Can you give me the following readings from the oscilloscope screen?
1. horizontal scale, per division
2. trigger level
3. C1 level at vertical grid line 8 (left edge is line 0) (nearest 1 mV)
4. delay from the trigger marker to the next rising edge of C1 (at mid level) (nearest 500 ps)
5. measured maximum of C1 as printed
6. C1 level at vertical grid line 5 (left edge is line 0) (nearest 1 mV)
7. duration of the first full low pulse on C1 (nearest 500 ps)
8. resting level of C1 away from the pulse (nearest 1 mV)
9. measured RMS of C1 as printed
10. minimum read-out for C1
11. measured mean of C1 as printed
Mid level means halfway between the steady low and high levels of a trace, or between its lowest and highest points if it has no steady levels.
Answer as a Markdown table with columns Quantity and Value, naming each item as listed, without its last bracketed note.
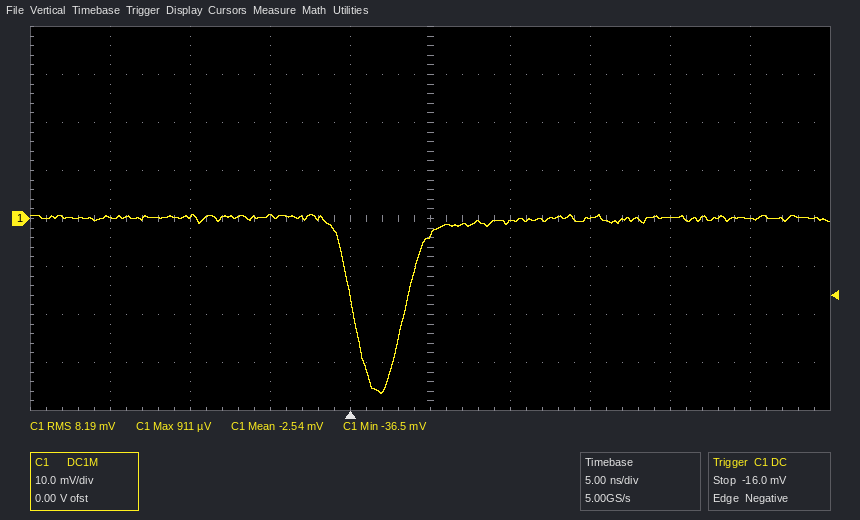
| Quantity | Value |
|---|---|
| horizontal scale, per division | 5 ns |
| trigger level | -16.0 mV |
| C1 level at vertical grid line 8 (left edge is line 0) | 0 mV |
| delay from the trigger marker to the next rising edge of C1 (at mid level) | 3.5 ns |
| measured maximum of C1 as printed | 911 µV |
| C1 level at vertical grid line 5 (left edge is line 0) | -3 mV |
| duration of the first full low pulse on C1 | 3.5 ns |
| resting level of C1 away from the pulse | 0 mV |
| measured RMS of C1 as printed | 8.19 mV |
| minimum read-out for C1 | -36.5 mV |
| measured mean of C1 as printed | -2.54 mV |
